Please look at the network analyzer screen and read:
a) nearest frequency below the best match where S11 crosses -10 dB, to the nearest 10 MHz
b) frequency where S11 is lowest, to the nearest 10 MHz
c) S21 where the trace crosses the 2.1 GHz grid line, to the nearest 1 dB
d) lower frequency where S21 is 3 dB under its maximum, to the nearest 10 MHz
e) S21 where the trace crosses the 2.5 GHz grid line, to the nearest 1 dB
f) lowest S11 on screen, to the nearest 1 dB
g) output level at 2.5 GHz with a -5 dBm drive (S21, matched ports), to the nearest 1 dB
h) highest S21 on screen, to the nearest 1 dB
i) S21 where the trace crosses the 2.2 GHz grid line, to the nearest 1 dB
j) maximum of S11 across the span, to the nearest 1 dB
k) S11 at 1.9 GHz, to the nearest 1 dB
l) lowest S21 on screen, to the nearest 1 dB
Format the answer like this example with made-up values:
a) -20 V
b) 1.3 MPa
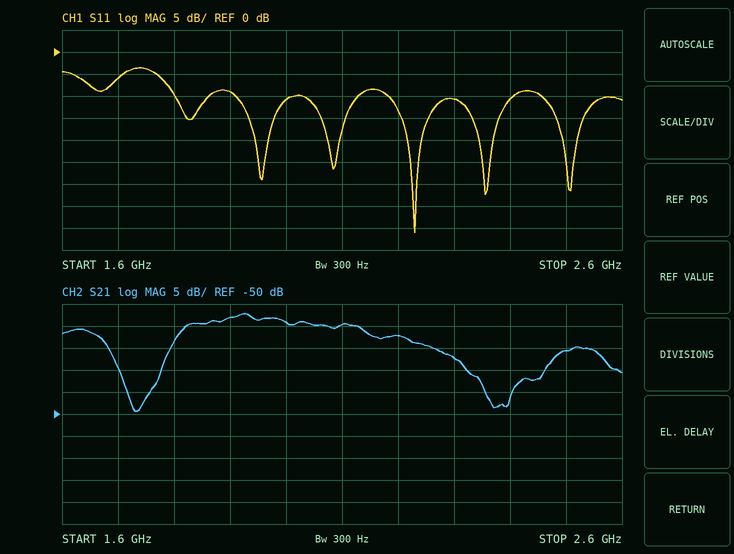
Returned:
a) 2.18 GHz
b) 2.23 GHz
c) -30 dB
d) 1.82 GHz
e) -36 dB
f) -41 dB
g) -41 dBm
h) -27 dB
i) -32 dB
j) -4 dB
k) -9 dB
l) -49 dB
